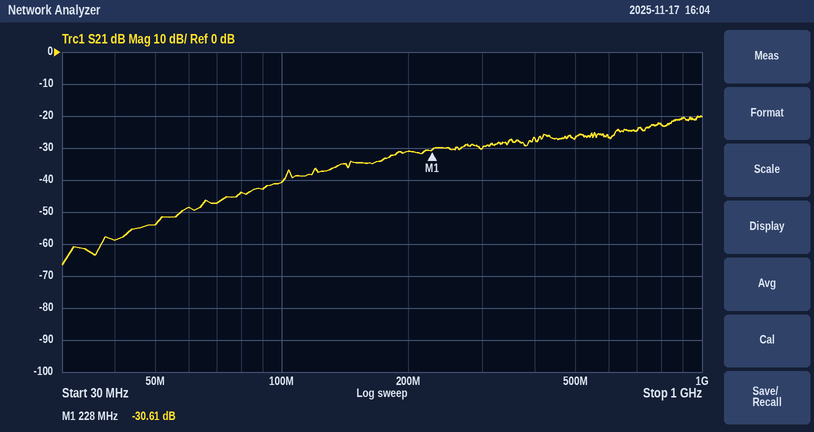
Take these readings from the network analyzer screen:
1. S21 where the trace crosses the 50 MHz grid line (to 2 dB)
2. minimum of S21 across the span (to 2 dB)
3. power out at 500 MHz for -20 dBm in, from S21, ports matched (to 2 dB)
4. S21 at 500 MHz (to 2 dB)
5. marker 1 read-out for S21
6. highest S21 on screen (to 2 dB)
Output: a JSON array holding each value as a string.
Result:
["-54 dB", "-66 dB", "-46 dBm", "-26 dB", "-30.61 dB", "-20 dB"]
